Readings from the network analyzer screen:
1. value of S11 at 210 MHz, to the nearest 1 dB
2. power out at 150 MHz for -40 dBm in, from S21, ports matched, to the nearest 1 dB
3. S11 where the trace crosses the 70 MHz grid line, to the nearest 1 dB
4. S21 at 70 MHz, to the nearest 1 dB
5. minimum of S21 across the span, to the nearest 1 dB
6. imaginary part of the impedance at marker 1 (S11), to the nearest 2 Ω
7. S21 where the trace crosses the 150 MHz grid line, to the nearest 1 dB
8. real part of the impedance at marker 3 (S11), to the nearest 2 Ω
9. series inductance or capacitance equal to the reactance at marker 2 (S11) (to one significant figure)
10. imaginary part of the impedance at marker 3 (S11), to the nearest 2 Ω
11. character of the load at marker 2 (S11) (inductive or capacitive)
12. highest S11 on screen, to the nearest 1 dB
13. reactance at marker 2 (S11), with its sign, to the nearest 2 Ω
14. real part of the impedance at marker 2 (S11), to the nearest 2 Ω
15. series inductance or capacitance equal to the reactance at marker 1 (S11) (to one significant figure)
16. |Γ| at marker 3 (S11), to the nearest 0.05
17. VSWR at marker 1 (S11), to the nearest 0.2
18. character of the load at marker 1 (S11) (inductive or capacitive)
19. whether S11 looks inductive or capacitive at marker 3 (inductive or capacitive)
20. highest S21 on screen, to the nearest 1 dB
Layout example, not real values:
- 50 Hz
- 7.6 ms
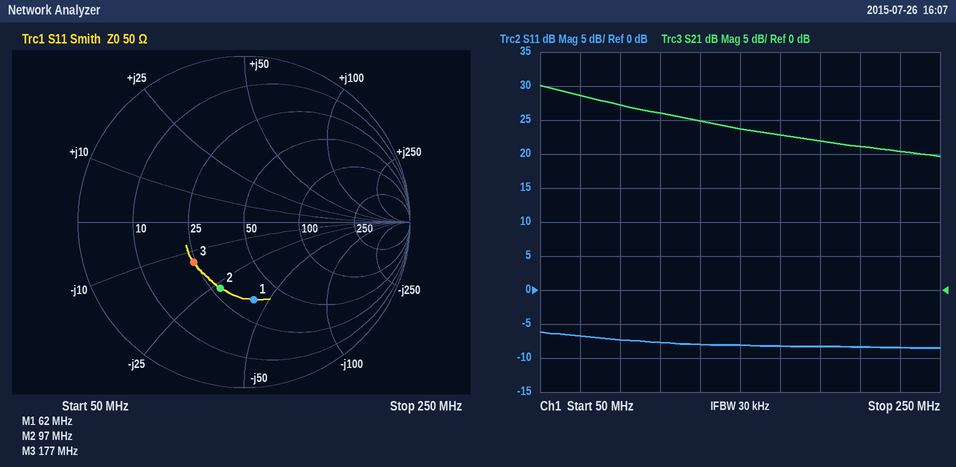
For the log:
- -8 dB
- -16 dBm
- -7 dB
- 29 dB
- 20 dB
- -42 Ω
- 24 dB
- 24 Ω
- 60 pF
- -14 Ω
- capacitive
- -6 dB
- -28 Ω
- 28 Ω
- 60 pF
- 0.40
- 2.8
- capacitive
- capacitive
- 30 dB
